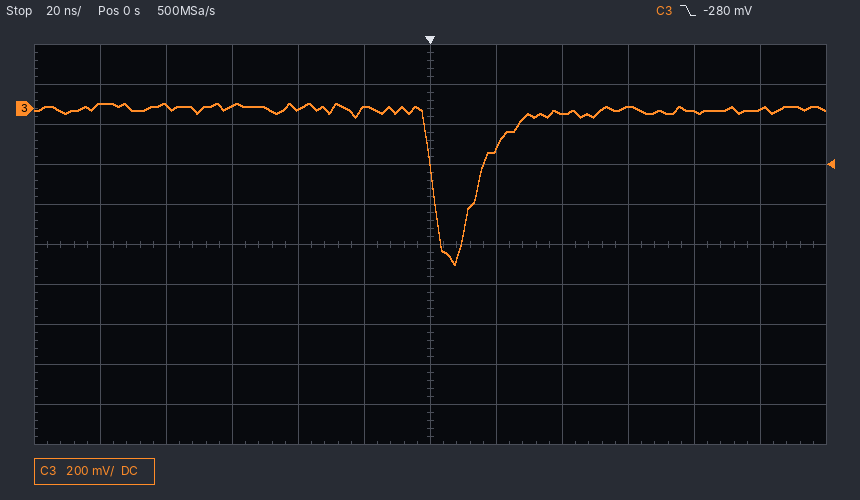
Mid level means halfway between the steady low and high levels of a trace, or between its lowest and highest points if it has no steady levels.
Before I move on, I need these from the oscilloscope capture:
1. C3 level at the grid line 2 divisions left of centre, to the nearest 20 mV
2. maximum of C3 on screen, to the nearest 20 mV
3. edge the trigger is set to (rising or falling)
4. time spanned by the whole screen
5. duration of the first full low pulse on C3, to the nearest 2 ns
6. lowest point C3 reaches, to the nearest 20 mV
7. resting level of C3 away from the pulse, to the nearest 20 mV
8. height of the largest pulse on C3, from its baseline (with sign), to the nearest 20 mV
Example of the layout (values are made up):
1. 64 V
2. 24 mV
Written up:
1. 0 mV
2. 20 mV
3. falling
4. 240 ns
5. 14 ns
6. -780 mV
7. 0 mV
8. -780 mV
